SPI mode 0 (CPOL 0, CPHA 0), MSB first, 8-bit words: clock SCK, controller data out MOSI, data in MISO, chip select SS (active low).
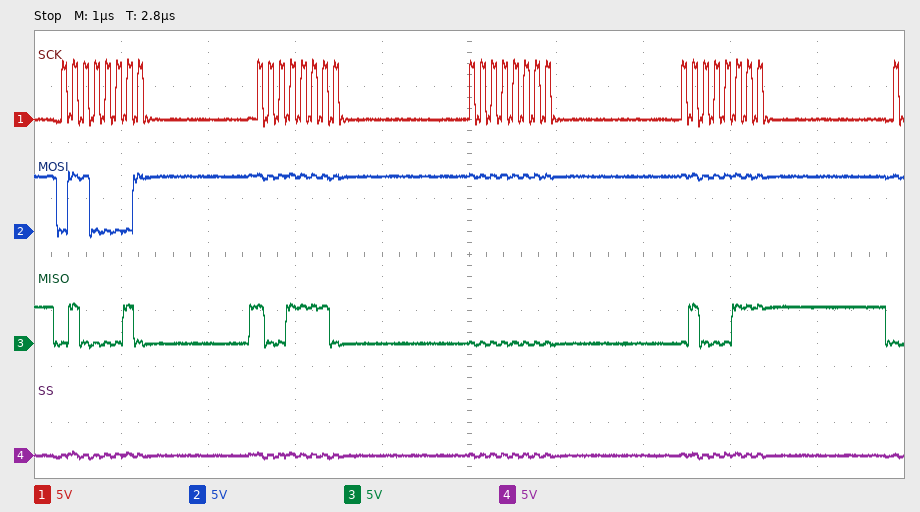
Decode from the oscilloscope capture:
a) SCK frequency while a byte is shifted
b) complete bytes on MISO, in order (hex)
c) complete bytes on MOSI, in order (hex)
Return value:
8 MHz
42 9E 00 47
61 FF FF FF
